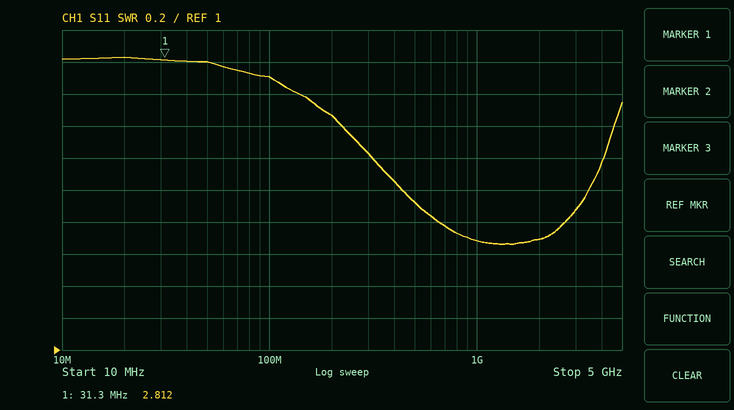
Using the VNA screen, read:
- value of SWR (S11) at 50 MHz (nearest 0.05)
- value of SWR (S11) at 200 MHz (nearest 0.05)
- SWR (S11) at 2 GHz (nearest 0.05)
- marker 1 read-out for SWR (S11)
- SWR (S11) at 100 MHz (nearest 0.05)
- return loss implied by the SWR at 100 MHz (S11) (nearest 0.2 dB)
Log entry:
2.80
2.45
1.70
2.812
2.70
6.8 dB
